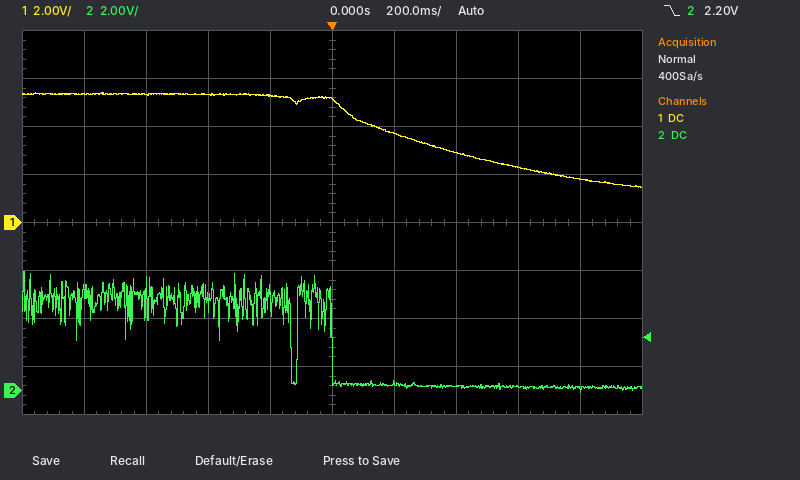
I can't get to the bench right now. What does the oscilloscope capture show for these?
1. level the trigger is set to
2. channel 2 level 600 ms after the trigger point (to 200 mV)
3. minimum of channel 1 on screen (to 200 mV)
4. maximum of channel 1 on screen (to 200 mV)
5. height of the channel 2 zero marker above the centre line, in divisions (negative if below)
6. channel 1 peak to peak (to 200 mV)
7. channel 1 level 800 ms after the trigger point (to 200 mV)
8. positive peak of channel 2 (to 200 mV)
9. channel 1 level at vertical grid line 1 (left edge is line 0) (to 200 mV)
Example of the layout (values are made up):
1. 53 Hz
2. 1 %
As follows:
1. 2.20 V
2. 200 mV
3. 1.4 V
4. 5.4 V
5. -3.5 div
6. 4.0 V
7. 1.8 V
8. 5.0 V
9. 5.4 V
